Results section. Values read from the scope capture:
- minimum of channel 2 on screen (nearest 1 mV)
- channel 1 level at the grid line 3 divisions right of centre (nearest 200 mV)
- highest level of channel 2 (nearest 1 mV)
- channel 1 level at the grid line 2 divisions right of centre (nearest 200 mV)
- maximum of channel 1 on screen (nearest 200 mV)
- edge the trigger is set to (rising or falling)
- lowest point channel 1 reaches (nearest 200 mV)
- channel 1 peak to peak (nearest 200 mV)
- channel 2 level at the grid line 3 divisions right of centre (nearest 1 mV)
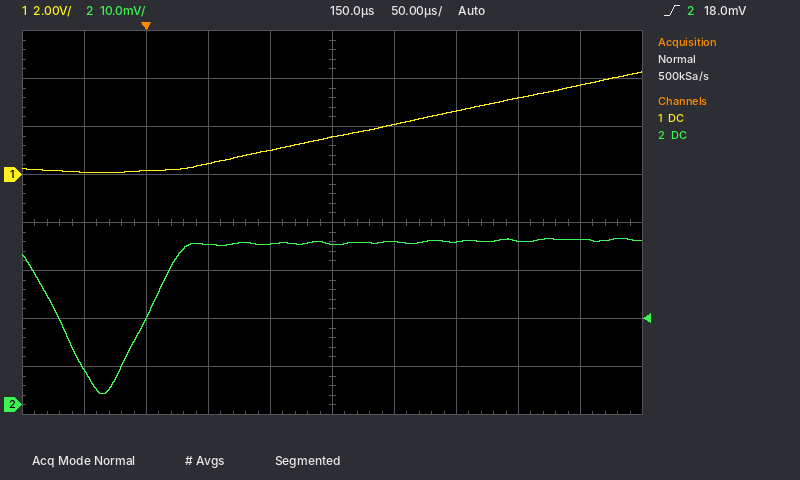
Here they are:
2 mV
3.2 V
35 mV
2.6 V
4.2 V
rising
0.0 V
4.2 V
34 mV
